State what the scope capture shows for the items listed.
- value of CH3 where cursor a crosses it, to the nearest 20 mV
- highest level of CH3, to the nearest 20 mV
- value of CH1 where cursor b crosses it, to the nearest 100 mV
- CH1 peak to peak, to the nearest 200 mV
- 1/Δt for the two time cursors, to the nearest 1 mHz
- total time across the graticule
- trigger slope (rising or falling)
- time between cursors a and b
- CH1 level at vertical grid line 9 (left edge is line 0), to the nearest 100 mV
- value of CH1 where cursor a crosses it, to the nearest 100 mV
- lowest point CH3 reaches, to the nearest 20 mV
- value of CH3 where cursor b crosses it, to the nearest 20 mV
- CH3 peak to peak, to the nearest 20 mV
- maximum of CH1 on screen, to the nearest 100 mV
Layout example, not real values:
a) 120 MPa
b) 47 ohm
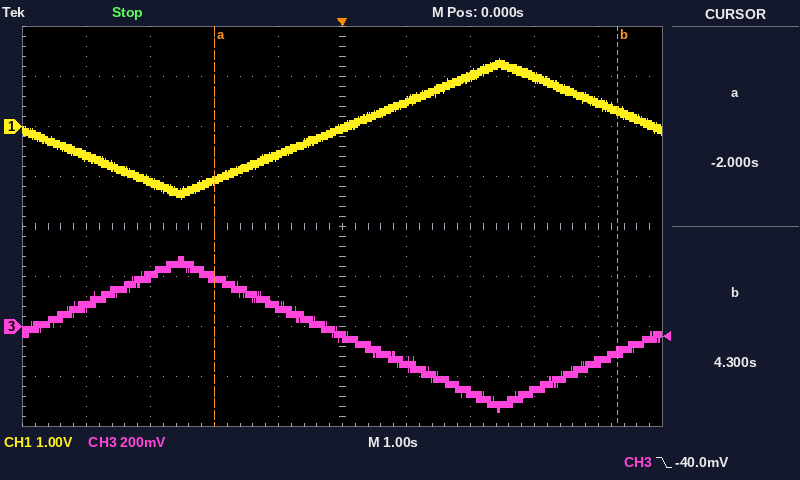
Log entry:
a) 200 mV
b) 280 mV
c) 300 mV
d) 2.8 V
e) 159 mHz
f) 10 s
g) falling
h) 6.3 s
i) 500 mV
j) -1.1 V
k) -340 mV
l) -100 mV
m) 620 mV
n) 1.4 V
